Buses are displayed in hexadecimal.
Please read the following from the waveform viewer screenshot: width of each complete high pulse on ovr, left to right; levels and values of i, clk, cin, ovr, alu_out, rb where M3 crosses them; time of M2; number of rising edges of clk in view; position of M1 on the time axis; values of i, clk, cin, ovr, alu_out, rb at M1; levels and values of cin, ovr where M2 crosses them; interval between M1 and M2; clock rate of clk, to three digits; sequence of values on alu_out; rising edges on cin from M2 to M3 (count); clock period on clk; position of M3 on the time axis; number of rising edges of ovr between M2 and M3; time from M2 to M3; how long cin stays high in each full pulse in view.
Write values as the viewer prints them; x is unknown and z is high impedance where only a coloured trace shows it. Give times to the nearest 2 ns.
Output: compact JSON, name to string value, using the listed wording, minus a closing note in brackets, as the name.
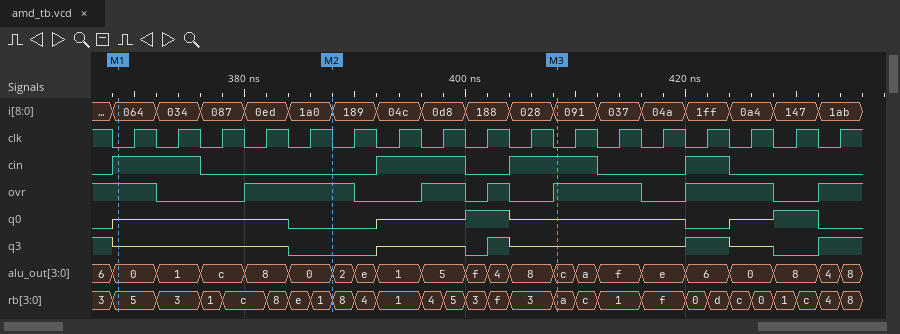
{"width of each complete high pulse on ovr, left to right": "10 ns, 4 ns, 2 ns, 8 ns, 8 ns", "levels and values of i, clk, cin, ovr, alu_out, rb where M3 crosses them": "i=091, clk=0, cin=1, ovr=1, alu_out=c, rb=a", "time of M2": "388 ns", "number of rising edges of clk in view": "17", "position of M1 on the time axis": "368 ns", "values of i, clk, cin, ovr, alu_out, rb at M1": "i=064, clk=0, cin=1, ovr=1, alu_out=0, rb=5", "levels and values of cin, ovr where M2 crosses them": "cin=0, ovr=1", "interval between M1 and M2": "20 ns", "clock rate of clk, to three digits": "250 MHz", "sequence of values on alu_out": "6, 0, 1, c, 8, 0, 2, e, 1, 5, f, 4, 8, c, a, f, e, 6, 0, 8, 4, 8", "rising edges on cin from M2 to M3": "2", "clock period on clk": "4 ns", "position of M3 on the time axis": "408 ns", "number of rising edges of ovr between M2 and M3": "3", "time from M2 to M3": "20 ns", "how long cin stays high in each full pulse in view": "8 ns, 8 ns, 8 ns, 4 ns"}
